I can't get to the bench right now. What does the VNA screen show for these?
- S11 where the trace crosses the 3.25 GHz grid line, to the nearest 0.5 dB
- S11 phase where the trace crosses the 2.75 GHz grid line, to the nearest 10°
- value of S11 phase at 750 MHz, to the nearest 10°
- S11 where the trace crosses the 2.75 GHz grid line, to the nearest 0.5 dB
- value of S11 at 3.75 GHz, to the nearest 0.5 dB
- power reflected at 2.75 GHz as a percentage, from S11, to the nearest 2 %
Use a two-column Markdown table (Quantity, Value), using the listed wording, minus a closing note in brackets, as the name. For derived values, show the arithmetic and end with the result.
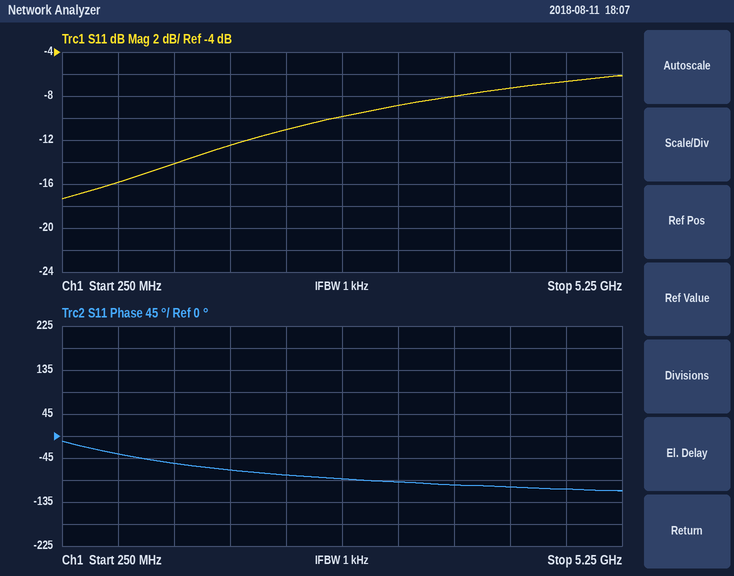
| Quantity | Value |
|---|---|
| S11 where the trace crosses the 3.25 GHz grid line, to the nearest 0.5 dB | -9.0 dB |
| S11 phase where the trace crosses the 2.75 GHz grid line, to the nearest 10° | -90° |
| value of S11 phase at 750 MHz, to the nearest 10° | -40° |
| S11 where the trace crosses the 2.75 GHz grid line, to the nearest 0.5 dB | -10.0 dB |
| value of S11 at 3.75 GHz, to the nearest 0.5 dB | -8.0 dB |
| power reflected at 2.75 GHz as a percentage, from S11, to the nearest 2 % | 10^(-10/10) ≈ 10 % |
